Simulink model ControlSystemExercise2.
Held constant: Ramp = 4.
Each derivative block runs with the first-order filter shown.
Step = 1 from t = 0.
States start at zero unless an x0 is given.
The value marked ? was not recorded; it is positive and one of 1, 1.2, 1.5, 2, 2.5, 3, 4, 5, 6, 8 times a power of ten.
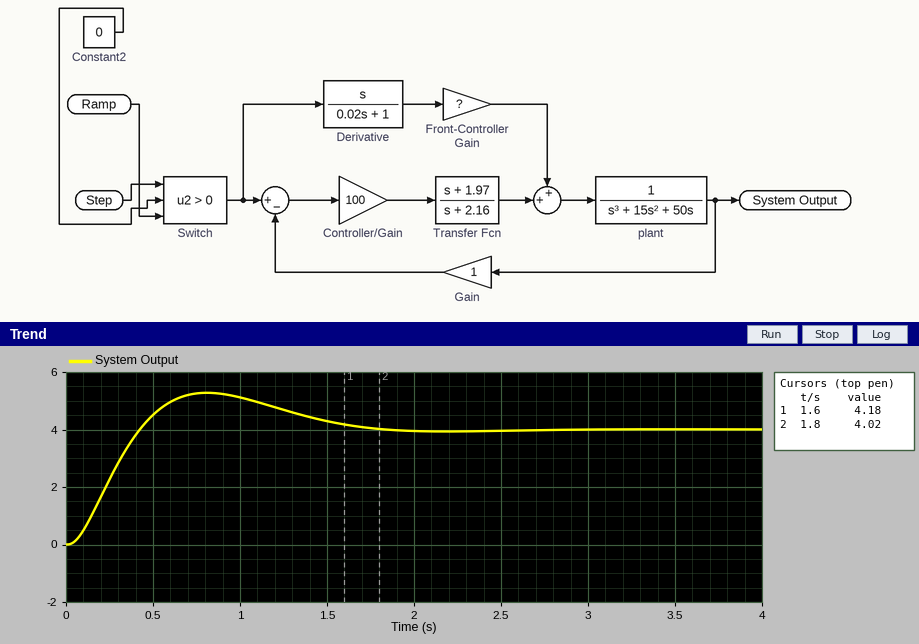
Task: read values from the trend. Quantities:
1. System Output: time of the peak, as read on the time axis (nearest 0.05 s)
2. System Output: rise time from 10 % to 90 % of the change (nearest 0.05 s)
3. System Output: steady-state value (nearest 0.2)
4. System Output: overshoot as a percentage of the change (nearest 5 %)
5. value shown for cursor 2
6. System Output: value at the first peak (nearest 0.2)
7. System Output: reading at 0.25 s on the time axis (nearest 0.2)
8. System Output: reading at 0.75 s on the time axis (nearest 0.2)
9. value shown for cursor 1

0.80 s
0.30 s
4.0
30 %
4.02
5.2
2.2
5.2
4.18
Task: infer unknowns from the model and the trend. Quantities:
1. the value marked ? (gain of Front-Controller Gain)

50
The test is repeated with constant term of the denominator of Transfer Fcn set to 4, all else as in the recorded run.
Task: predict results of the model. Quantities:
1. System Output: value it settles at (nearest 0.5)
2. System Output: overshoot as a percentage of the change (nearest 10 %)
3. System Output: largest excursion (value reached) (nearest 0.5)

4.0
20 %
5.0
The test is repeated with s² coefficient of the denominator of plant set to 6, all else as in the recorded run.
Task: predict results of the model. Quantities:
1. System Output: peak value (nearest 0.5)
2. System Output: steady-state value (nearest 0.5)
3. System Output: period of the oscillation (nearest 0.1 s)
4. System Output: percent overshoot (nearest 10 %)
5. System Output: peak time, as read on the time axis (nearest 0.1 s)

6.5
4.0
1.0 s
60 %
0.5 s
